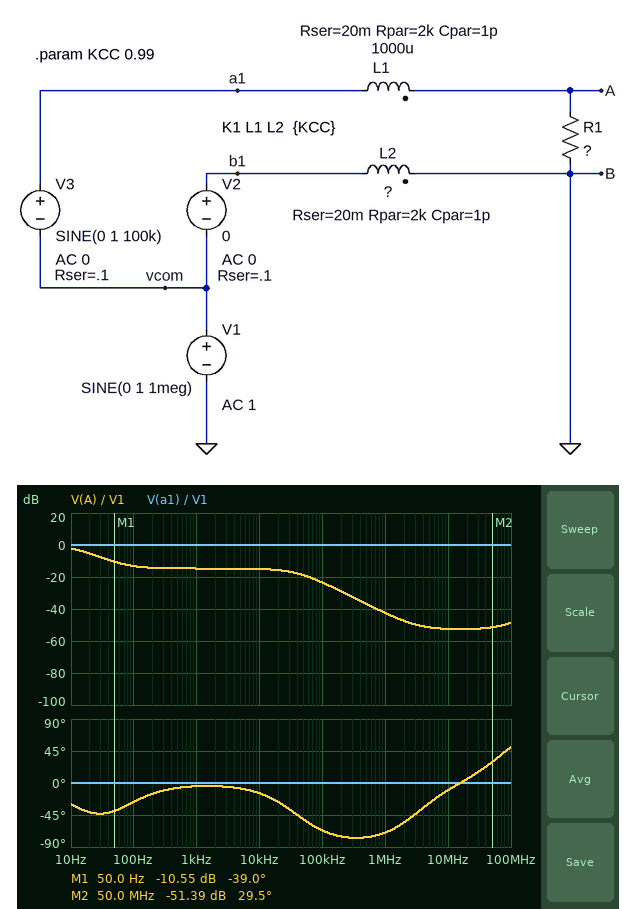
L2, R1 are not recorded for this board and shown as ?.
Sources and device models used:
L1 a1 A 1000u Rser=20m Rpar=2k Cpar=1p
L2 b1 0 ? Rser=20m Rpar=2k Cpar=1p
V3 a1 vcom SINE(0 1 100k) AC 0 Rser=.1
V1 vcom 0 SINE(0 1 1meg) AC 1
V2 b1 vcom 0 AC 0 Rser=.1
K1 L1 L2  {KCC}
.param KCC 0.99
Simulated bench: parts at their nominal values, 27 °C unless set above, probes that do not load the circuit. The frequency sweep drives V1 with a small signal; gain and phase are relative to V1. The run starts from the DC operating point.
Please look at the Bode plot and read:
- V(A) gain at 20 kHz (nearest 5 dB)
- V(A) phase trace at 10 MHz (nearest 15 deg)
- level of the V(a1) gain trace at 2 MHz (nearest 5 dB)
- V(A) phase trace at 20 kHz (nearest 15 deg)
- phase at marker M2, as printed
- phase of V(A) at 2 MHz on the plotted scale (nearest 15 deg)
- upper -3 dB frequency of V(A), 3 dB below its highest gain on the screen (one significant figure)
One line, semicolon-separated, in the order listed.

-15 dB; -15 deg; 0 dB; -30 deg; 29.5 deg; -60 deg; 20 Hz
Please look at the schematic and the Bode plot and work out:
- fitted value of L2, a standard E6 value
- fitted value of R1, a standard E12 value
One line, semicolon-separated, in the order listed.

1.5 mH; 4.7 Ω
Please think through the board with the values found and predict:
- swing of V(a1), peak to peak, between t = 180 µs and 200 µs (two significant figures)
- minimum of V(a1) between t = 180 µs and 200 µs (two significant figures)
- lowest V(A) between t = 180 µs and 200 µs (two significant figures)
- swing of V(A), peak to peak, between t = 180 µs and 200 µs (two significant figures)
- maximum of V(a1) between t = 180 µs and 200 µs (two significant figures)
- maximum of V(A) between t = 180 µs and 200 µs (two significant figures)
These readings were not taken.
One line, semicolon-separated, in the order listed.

4.0 V; -2.0 V; -350 mV; 700 mV; 2.0 V; 360 mV
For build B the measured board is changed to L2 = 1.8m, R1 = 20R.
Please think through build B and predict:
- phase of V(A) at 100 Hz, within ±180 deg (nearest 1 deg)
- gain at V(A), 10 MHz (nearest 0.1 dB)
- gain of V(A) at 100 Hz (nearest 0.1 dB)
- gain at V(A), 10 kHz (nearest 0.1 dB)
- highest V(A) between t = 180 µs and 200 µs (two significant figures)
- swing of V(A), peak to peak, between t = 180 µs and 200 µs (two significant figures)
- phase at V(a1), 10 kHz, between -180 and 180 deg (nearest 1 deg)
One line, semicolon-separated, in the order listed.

-16 deg; -39.7 dB; -11.1 dB; -11.7 dB; 880 mV; 1.7 V; 0 deg
